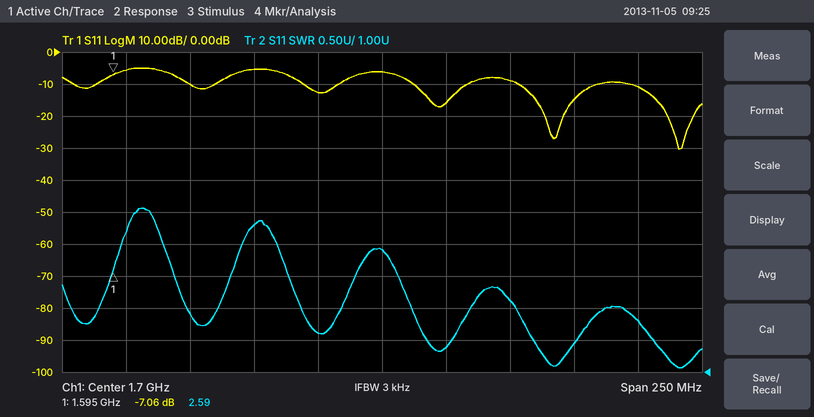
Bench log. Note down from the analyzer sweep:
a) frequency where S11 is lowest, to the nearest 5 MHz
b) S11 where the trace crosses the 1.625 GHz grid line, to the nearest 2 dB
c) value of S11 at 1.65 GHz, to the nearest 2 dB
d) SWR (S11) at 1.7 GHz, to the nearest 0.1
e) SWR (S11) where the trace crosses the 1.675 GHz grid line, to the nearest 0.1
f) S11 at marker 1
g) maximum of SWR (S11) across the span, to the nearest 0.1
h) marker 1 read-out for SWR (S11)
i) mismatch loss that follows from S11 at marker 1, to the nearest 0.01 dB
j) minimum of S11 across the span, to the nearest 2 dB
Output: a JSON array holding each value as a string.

["1.815 GHz", "-10 dB", "-6 dB", "2.9", "1.6", "-7.06 dB", "3.6", "2.59", "0.95 dB", "-30 dB"]
